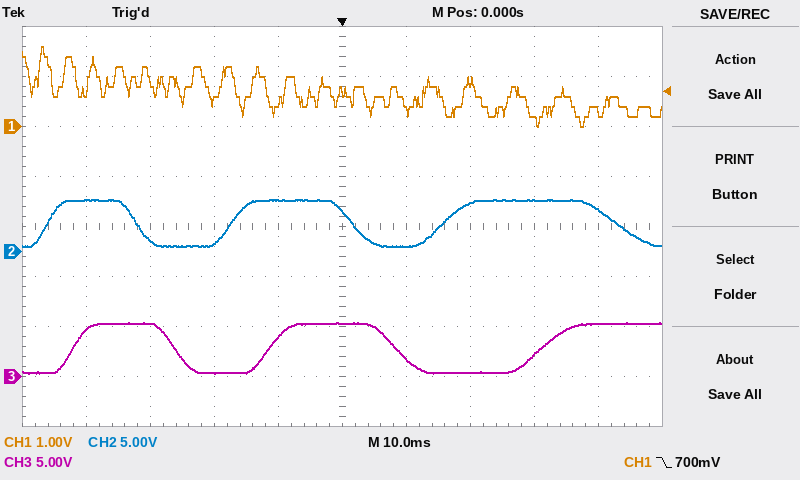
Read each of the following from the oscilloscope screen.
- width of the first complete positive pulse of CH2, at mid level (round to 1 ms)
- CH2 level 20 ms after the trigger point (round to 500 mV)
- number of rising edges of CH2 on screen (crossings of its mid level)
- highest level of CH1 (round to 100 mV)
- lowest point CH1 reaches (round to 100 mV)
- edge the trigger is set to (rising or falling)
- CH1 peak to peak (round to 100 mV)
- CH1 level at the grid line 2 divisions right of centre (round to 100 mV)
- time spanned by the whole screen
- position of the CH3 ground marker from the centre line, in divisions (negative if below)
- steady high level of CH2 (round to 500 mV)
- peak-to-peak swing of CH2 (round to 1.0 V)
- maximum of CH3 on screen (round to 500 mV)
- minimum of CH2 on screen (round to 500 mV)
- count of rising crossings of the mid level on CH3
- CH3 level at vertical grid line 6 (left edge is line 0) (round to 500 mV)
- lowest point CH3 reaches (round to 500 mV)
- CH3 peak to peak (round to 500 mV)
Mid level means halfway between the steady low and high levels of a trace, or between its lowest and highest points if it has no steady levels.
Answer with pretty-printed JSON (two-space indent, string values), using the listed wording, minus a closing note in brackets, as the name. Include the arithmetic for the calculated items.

{
  "width of the first complete positive pulse of CH2, at mid level": "14 ms",
  "CH2 level 20 ms after the trigger point": "5.0 V",
  "number of rising edges of CH2 on screen": "3",
  "highest level of CH1": "1.6 V",
  "lowest point CH1 reaches": "0.0 V",
  "edge the trigger is set to": "falling",
  "CH1 peak to peak": "1.6 V − (0.0 V) = 1.6 V",
  "CH1 level at the grid line 2 divisions right of centre": "900 mV",
  "time spanned by the whole screen": "100 ms",
  "position of the CH3 ground marker from the centre line, in divisions": "-3.0 div",
  "steady high level of CH2": "5.0 V",
  "peak-to-peak swing of CH2": "5.0 V",
  "maximum of CH3 on screen": "5.5 V",
  "minimum of CH2 on screen": "500 mV",
  "count of rising crossings of the mid level on CH3": "3",
  "CH3 level at vertical grid line 6 (left edge is line 0)": "2.0 V",
  "lowest point CH3 reaches": "500 mV",
  "CH3 peak to peak": "5.5 V − (500 mV) = 5.0 V"
}
